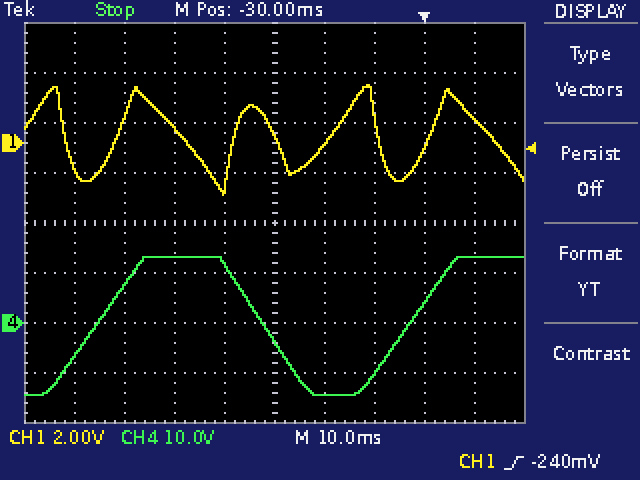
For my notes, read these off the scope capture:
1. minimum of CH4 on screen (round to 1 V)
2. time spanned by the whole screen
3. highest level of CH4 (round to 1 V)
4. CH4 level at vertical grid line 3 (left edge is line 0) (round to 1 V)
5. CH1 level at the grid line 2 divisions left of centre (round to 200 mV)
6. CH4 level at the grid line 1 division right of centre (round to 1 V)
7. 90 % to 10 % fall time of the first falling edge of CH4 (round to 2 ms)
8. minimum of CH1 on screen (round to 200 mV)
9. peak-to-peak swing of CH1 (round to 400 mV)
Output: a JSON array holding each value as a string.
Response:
["-14 V", "100 ms", "13 V", "13 V", "600 mV", "-14 V", "14 ms", "-2.0 V", "4.4 V"]
